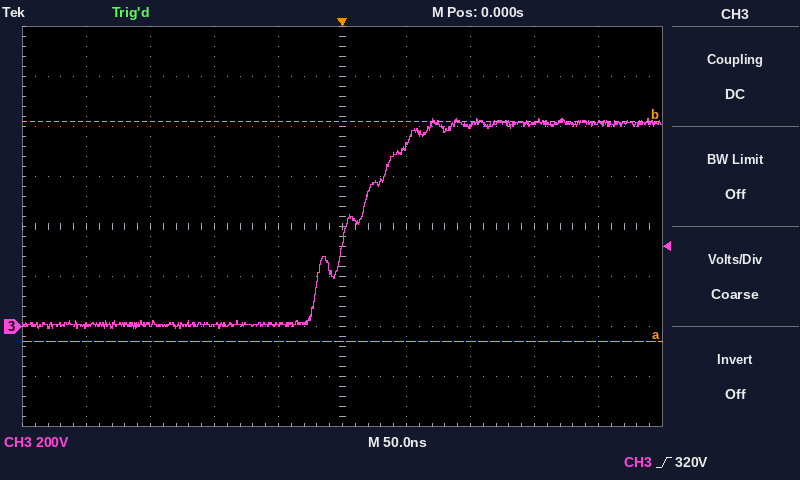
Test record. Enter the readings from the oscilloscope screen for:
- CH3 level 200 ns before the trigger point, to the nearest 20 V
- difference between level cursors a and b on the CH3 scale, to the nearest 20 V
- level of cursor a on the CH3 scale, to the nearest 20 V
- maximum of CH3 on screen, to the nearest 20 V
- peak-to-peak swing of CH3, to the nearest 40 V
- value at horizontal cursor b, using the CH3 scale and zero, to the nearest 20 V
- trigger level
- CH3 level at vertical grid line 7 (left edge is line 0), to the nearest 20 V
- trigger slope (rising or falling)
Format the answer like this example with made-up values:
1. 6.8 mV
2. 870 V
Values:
1. 0 V
2. 880 V
3. -60 V
4. 840 V
5. 840 V
6. 820 V
7. 320 V
8. 800 V
9. rising
